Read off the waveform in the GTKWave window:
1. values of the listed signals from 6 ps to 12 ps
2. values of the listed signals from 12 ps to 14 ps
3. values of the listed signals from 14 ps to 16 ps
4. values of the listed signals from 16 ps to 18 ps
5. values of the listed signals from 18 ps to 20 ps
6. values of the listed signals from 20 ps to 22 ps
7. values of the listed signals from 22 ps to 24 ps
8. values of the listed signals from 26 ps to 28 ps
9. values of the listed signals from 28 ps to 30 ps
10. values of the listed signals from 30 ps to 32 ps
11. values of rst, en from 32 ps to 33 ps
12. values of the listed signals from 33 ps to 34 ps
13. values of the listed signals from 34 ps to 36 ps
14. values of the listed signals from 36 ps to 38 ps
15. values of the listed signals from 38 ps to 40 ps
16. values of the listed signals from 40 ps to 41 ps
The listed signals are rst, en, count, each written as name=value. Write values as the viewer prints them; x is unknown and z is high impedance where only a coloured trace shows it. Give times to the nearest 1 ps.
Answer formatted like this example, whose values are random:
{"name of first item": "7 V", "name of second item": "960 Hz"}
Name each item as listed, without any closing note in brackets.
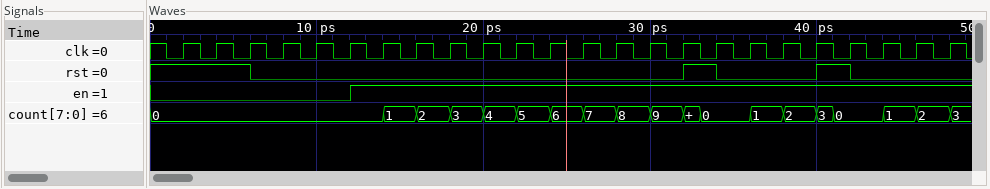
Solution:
{"values of the listed signals from 6 ps to 12 ps": "rst=0, en=0, count=0", "values of the listed signals from 12 ps to 14 ps": "rst=0, en=1, count=0", "values of the listed signals from 14 ps to 16 ps": "rst=0, en=1, count=1", "values of the listed signals from 16 ps to 18 ps": "rst=0, en=1, count=2", "values of the listed signals from 18 ps to 20 ps": "rst=0, en=1, count=3", "values of the listed signals from 20 ps to 22 ps": "rst=0, en=1, count=4", "values of the listed signals from 22 ps to 24 ps": "rst=0, en=1, count=5", "values of the listed signals from 26 ps to 28 ps": "rst=0, en=1, count=7", "values of the listed signals from 28 ps to 30 ps": "rst=0, en=1, count=8", "values of the listed signals from 30 ps to 32 ps": "rst=0, en=1, count=9", "values of rst, en from 32 ps to 33 ps": "rst=1, en=1", "values of the listed signals from 33 ps to 34 ps": "rst=1, en=1, count=0", "values of the listed signals from 34 ps to 36 ps": "rst=0, en=1, count=0", "values of the listed signals from 36 ps to 38 ps": "rst=0, en=1, count=1", "values of the listed signals from 38 ps to 40 ps": "rst=0, en=1, count=2", "values of the listed signals from 40 ps to 41 ps": "rst=1, en=1, count=3"}
